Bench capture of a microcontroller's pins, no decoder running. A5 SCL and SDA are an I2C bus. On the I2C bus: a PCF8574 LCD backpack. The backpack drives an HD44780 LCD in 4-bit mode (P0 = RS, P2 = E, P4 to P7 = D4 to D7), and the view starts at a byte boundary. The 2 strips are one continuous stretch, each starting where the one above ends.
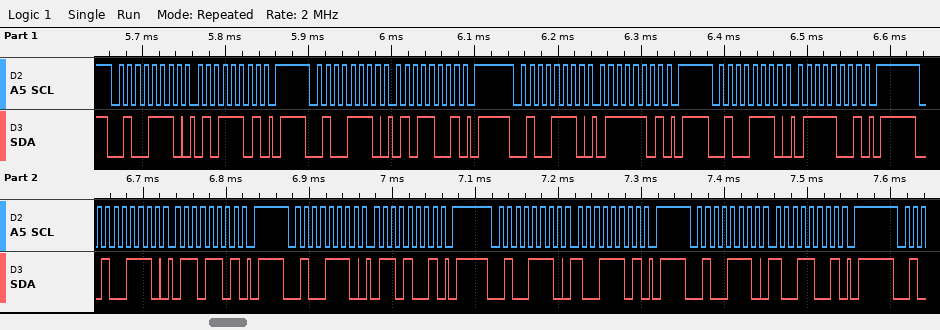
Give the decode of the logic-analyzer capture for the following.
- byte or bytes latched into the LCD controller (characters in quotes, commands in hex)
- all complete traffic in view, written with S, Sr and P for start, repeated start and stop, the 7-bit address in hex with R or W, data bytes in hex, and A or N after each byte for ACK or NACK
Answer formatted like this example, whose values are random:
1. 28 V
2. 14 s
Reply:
1. 'W' 'i'
2. S 27W A 5D A P S 27W A 59 A P S 27W A 7D A P S 27W A 79 A P S 27W A 6D A P S 27W A 69 A P S 27W A 9D A P S 27W A 99 A P
